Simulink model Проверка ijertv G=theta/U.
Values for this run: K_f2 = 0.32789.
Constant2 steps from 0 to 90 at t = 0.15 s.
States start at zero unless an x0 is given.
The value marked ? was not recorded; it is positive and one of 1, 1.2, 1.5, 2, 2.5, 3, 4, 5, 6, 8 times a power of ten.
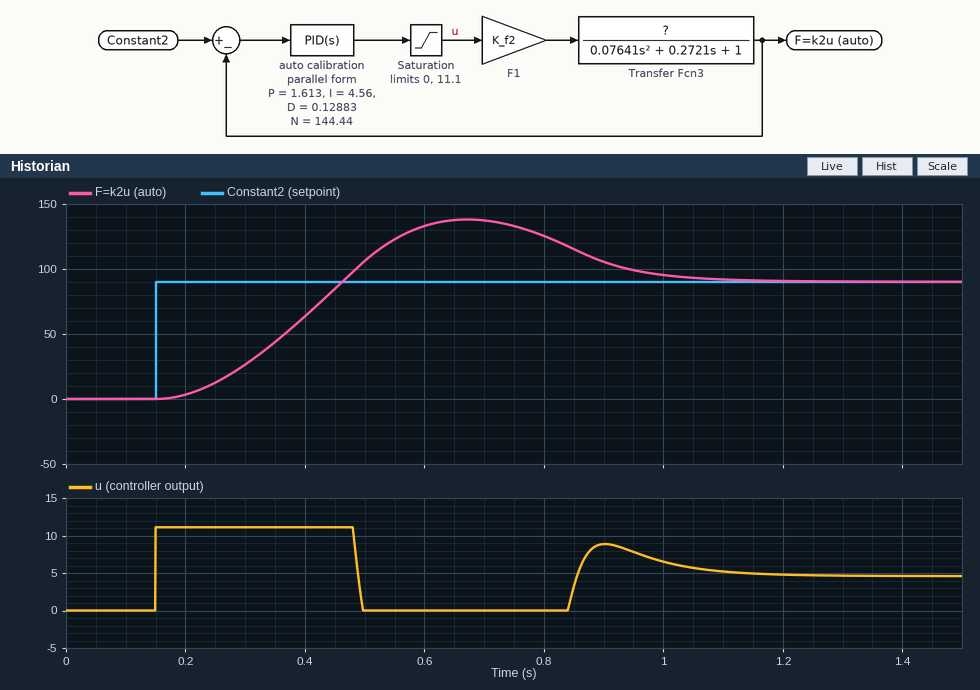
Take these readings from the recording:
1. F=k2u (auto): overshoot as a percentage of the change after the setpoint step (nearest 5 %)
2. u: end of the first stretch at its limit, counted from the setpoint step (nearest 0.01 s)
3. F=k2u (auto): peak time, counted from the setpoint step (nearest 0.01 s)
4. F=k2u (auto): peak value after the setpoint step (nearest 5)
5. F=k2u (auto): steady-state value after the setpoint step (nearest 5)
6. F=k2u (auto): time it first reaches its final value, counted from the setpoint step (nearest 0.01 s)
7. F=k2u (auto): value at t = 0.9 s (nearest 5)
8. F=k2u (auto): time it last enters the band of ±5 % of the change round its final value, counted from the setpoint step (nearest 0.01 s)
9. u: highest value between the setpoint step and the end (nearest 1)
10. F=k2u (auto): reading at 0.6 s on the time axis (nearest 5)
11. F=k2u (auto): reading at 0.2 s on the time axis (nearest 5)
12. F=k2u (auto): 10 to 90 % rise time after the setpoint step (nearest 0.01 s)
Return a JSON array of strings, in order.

["55 %", "0.33 s", "0.52 s", "140", "90", "0.31 s", "105", "0.87 s", "11", "135", "5", "0.21 s"]
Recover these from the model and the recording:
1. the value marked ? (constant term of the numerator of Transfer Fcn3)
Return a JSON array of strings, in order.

["60"]
